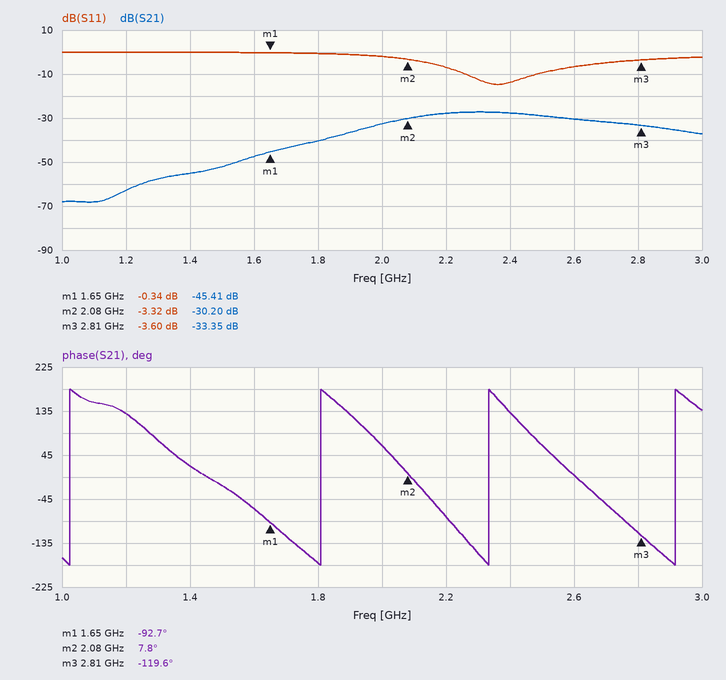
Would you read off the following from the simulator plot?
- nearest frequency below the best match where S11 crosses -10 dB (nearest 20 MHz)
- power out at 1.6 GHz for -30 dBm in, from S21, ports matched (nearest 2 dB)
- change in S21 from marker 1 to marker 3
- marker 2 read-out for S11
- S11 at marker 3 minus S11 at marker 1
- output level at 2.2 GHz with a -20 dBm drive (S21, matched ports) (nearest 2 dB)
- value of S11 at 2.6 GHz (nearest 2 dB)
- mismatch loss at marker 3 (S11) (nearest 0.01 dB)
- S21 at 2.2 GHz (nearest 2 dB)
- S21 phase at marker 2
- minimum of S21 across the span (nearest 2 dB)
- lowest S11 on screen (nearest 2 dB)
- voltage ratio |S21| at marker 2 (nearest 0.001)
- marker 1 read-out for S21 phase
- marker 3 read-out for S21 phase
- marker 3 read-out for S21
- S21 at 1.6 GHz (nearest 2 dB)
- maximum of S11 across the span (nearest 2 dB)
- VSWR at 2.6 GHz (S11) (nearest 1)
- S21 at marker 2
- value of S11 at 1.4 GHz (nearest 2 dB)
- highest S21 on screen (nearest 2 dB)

2.26 GHz
-78 dBm
12.06 dB
-3.32 dB
-3.26 dB
-48 dBm
-6 dB
2.49 dB
-28 dB
7.8°
-68 dB
-14 dB
0.031
-92.7°
-119.6°
-33.35 dB
-48 dB
0 dB
3
-30.20 dB
0 dB
-28 dB
